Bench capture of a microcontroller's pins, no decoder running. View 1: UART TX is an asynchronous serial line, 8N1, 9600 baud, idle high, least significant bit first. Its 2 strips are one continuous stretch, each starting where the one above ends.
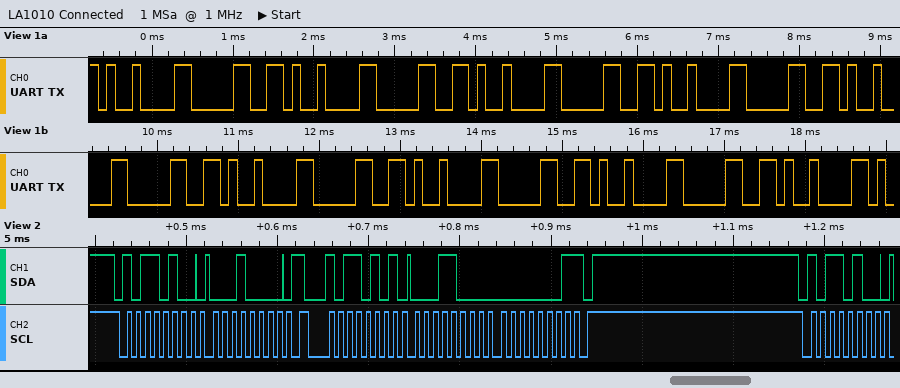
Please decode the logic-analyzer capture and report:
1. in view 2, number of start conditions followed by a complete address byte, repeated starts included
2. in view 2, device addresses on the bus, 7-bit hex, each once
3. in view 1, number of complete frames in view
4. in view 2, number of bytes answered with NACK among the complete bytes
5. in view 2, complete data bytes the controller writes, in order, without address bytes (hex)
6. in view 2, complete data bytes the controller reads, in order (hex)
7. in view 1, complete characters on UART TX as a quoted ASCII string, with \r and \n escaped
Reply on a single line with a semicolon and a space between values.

3; 0x5A; 17; 1; 10; 18 01; "\t0\t0\t0\t0\t0\t0\t0\t0\t"
